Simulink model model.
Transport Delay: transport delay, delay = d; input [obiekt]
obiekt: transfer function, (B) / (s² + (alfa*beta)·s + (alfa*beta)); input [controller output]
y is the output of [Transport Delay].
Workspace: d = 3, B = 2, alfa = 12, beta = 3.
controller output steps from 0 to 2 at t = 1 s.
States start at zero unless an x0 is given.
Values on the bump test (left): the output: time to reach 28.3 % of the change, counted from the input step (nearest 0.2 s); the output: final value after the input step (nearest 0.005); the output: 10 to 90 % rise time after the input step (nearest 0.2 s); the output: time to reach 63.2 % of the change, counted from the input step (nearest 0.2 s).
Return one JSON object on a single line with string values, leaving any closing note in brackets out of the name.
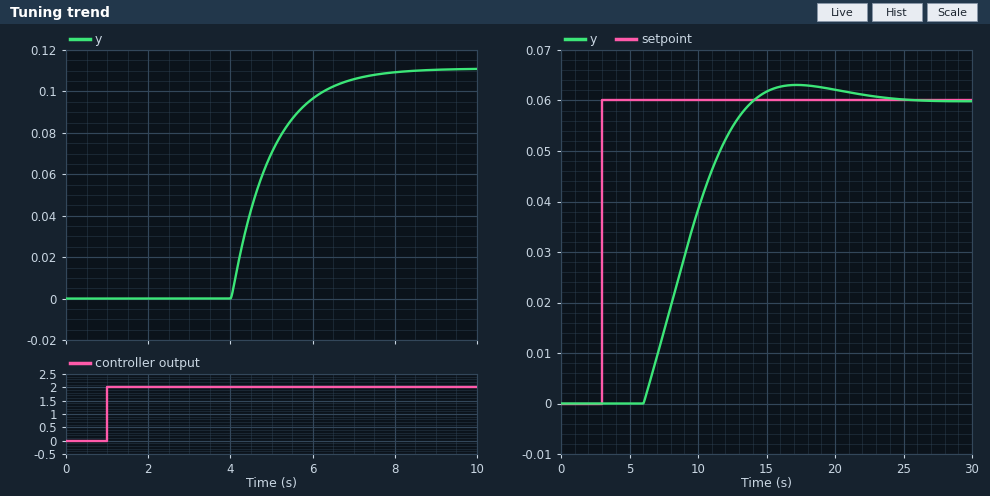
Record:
{"the output: time to reach 28.3 % of the change, counted from the input step": "3.4 s", "the output: final value after the input step": "0.110", "the output: 10 to 90 % rise time after the input step": "2.2 s", "the output: time to reach 63.2 % of the change, counted from the input step": "4.0 s"}
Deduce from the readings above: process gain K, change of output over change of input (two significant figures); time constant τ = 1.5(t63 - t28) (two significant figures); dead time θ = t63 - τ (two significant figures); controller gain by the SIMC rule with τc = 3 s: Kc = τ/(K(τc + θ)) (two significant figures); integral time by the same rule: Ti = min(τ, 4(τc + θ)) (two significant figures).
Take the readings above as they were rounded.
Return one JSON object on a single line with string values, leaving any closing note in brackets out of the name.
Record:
{"process gain K, change of output over change of input": "0.055", "time constant τ = 1.5(t63 - t28)": "0.90 s", "dead time θ = t63 - τ": "3.1 s", "controller gain by the SIMC rule with τc = 3 s: Kc = τ/(K(τc + θ))": "2.7", "integral time by the same rule: Ti = min(τ, 4(τc + θ))": "0.90 s"}
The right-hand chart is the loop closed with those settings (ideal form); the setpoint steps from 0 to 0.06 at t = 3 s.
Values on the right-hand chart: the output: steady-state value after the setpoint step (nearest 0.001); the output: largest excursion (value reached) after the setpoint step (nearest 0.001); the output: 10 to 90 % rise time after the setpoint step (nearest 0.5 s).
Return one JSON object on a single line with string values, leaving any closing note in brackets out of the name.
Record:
{"the output: steady-state value after the setpoint step": "0.060", "the output: largest excursion (value reached) after the setpoint step": "0.063", "the output: 10 to 90 % rise time after the setpoint step": "5.5 s"}
